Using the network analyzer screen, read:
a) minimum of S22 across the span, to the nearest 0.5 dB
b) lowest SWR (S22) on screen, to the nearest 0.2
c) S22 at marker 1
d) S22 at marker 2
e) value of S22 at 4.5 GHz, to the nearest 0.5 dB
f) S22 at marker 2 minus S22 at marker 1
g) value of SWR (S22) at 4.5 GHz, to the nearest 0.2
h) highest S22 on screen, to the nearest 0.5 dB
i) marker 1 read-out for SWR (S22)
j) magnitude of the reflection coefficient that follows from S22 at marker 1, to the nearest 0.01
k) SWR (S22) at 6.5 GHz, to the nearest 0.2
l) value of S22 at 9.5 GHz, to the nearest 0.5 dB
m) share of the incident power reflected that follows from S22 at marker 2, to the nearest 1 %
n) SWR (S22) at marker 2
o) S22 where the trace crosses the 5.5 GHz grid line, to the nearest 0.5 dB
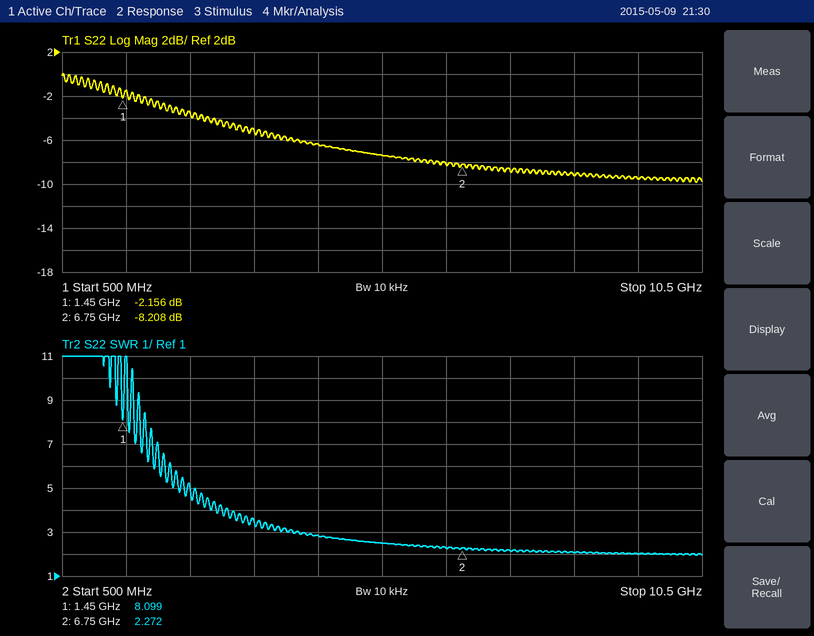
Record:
-10.0 dB
2.0
-2.156 dB
-8.208 dB
-6.5 dB
-6.052 dB
2.8
0.0 dB
8.099
0.78
2.2
-9.5 dB
15 %
2.272
-7.5 dB
